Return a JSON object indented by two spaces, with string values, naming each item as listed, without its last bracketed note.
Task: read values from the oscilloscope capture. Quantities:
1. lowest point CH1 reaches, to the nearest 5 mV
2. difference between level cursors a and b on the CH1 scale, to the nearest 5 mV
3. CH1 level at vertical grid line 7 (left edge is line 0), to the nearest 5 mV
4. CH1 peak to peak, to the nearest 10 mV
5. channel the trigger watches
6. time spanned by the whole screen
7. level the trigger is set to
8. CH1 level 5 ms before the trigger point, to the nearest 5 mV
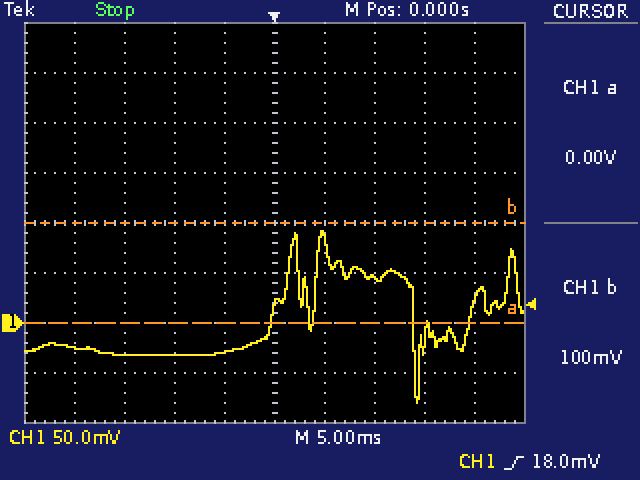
{
  "lowest point CH1 reaches, to the nearest 5 mV": "-80 mV",
  "difference between level cursors a and b on the CH1 scale, to the nearest 5 mV": "100 mV",
  "CH1 level at vertical grid line 7 (left edge is line 0), to the nearest 5 mV": "45 mV",
  "CH1 peak to peak, to the nearest 10 mV": "170 mV",
  "channel the trigger watches": "CH1",
  "time spanned by the whole screen": "50 ms",
  "level the trigger is set to": "18.0 mV",
  "CH1 level 5 ms before the trigger point, to the nearest 5 mV": "-30 mV"
}
